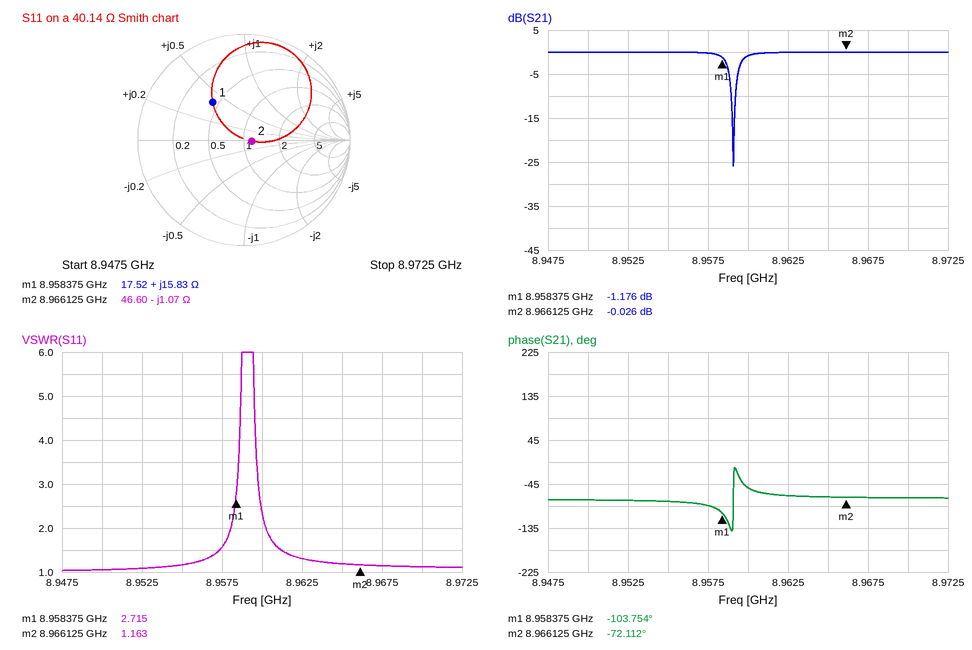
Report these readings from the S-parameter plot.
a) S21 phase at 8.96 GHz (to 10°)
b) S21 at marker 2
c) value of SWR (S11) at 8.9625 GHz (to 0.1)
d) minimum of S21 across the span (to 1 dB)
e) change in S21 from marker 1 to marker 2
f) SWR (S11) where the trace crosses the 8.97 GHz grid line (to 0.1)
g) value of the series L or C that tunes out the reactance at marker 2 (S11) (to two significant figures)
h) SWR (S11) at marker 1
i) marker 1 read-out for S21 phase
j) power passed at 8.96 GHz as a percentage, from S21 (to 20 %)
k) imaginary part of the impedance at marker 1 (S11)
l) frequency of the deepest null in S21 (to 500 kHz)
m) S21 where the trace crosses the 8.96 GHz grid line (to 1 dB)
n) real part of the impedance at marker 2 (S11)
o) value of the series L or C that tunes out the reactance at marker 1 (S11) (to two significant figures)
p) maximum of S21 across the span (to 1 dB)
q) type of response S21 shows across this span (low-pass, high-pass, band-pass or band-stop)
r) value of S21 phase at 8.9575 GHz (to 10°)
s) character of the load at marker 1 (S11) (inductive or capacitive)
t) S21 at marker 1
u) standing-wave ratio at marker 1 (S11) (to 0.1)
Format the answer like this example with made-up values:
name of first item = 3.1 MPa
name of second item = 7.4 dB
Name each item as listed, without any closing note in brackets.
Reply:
S21 phase at 8.96 GHz = -50°
S21 at marker 2 = -0.026 dB
value of SWR (S11) at 8.9625 GHz = 1.3
minimum of S21 across the span = -26 dB
change in S21 from marker 1 to marker 2 = 1.150 dB
SWR (S11) where the trace crosses the 8.97 GHz grid line = 1.1
value of the series L or C that tunes out the reactance at marker 2 (S11) = 19 pH
SWR (S11) at marker 1 = 2.715
marker 1 read-out for S21 phase = -103.754°
power passed at 8.96 GHz as a percentage, from S21 = 80 %
imaginary part of the impedance at marker 1 = +15.83 Ω
frequency of the deepest null in S21 = 8.9590 GHz
S21 where the trace crosses the 8.96 GHz grid line = -1 dB
real part of the impedance at marker 2 = 46.60 Ω
value of the series L or C that tunes out the reactance at marker 1 (S11) = 1.1 pF
maximum of S21 across the span = 0 dB
type of response S21 shows across this span = band-stop
value of S21 phase at 8.9575 GHz = -90°
character of the load at marker 1 (S11) = inductive
S21 at marker 1 = -1.176 dB
standing-wave ratio at marker 1 (S11) = 2.7
